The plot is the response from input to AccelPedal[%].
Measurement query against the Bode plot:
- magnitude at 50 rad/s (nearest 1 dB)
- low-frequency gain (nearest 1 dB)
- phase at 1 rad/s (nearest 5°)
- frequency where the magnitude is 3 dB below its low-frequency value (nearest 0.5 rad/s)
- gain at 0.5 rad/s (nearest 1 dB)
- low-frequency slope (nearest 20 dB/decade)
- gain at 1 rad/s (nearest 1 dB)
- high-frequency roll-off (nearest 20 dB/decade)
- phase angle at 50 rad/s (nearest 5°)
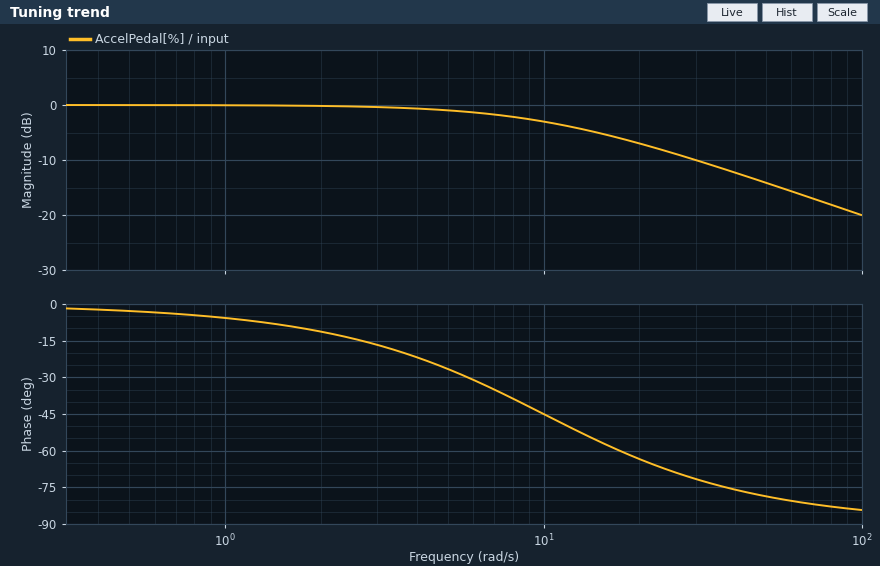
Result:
-14 dB
0 dB
-5°
10.0 rad/s
0 dB
0 dB/decade
0 dB
-20 dB/decade
-80°
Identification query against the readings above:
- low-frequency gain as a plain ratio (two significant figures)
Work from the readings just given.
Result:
1.0
